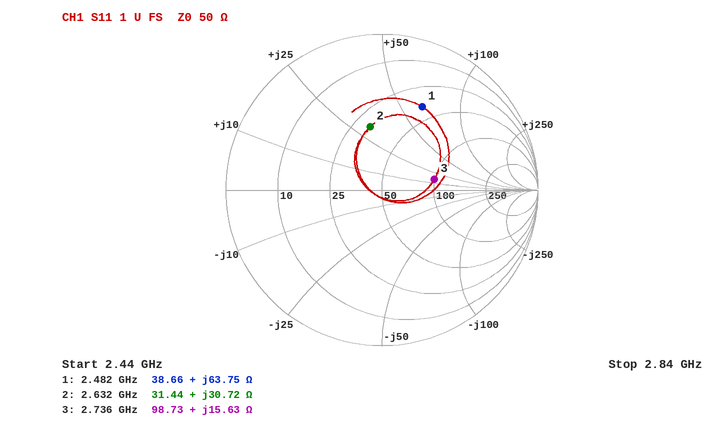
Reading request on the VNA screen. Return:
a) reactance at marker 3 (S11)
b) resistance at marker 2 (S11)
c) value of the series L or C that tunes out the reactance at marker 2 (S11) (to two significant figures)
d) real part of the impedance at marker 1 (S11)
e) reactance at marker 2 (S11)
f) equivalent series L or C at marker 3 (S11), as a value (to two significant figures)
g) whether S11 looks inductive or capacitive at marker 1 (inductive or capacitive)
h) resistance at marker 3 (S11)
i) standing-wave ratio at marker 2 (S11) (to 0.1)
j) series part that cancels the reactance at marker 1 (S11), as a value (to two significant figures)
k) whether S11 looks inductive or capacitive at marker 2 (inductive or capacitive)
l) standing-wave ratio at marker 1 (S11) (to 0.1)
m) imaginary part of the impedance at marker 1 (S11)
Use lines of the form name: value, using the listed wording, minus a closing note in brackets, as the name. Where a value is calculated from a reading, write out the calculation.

reactance at marker 3: +15.63 Ω
resistance at marker 2: 31.44 Ω
value of the series L or C that tunes out the reactance at marker 2 (S11): C = 1/(2π × 2.632 GHz × 30.72 Ω) ≈ 2.0 pF
real part of the impedance at marker 1: 38.66 Ω
reactance at marker 2: +30.72 Ω
equivalent series L or C at marker 3 (S11), as a value: L = 15.63 Ω/(2π × 2.736 GHz) ≈ 909 pH, so 910 pH to two significant figures
whether S11 looks inductive or capacitive at marker 1: inductive
resistance at marker 3: 98.73 Ω
standing-wave ratio at marker 2 (S11): 2.4
series part that cancels the reactance at marker 1 (S11), as a value: C = 1/(2π × 2.482 GHz × 63.75 Ω) ≈ 1.0 pF
whether S11 looks inductive or capacitive at marker 2: inductive
standing-wave ratio at marker 1 (S11): 3.9
imaginary part of the impedance at marker 1: +63.75 Ω
